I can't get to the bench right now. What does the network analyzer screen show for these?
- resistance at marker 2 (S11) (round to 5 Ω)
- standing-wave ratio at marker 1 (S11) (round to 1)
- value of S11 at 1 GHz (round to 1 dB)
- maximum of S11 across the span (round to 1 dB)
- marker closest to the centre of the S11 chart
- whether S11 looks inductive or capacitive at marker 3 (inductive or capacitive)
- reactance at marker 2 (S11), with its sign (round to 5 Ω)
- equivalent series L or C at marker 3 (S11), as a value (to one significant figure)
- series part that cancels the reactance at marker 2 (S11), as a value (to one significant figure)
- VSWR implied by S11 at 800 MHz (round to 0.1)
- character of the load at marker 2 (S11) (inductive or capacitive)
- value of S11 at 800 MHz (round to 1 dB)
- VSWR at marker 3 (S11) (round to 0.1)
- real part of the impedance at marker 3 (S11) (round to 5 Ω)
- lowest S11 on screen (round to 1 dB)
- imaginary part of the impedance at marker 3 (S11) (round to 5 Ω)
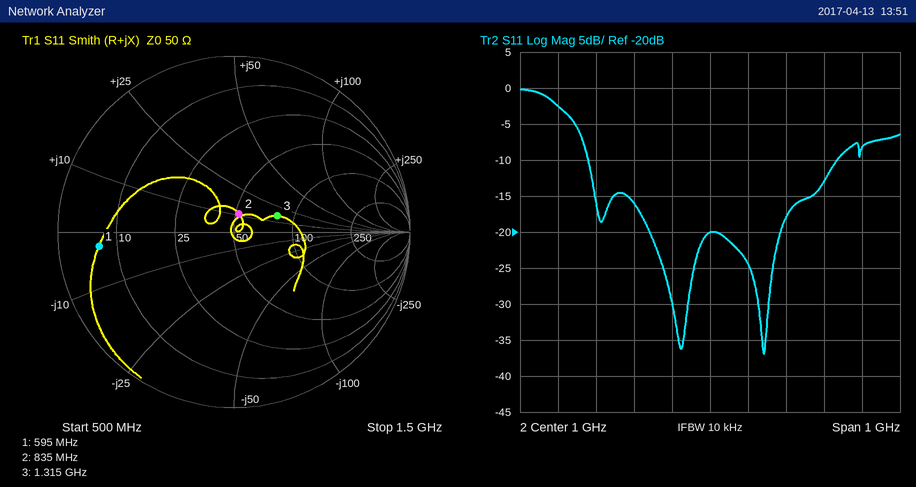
50 Ω
8
-20 dB
0 dB
marker 2
inductive
+10 Ω
2 nH
20 pF
1.4
inductive
-16 dB
1.7
80 Ω
-37 dB
+15 Ω
